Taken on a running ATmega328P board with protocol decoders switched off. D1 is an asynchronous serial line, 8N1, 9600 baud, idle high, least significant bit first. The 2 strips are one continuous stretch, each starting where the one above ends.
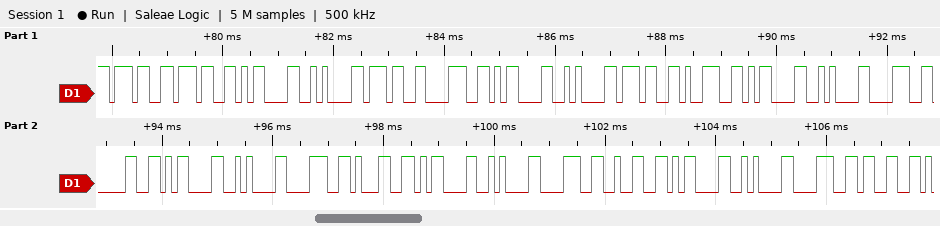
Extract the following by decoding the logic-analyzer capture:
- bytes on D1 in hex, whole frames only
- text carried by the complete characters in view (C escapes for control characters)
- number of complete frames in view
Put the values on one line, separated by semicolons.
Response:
37 37 0D 0A 37 38 0D 0A 37 39 0D 0A 38 30 0D 0A 38 31 0D 0A 38 32 0D 0A 38 33; "77\r\n78\r\n79\r\n80\r\n81\r\n82\r\n83"; 26
